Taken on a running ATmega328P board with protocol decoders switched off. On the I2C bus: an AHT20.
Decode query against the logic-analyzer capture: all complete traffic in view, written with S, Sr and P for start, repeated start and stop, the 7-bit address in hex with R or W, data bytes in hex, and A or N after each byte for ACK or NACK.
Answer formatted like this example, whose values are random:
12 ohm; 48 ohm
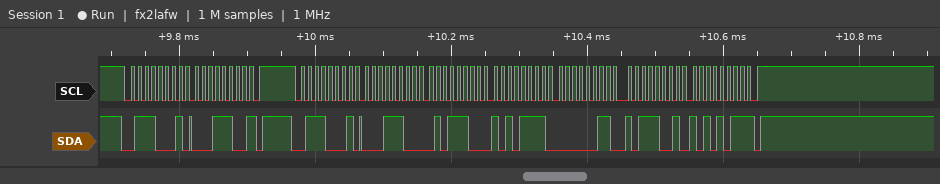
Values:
S 38R A 1C N P S 38R A 1C A 5C A AF A 03 A B9 A AB N P
